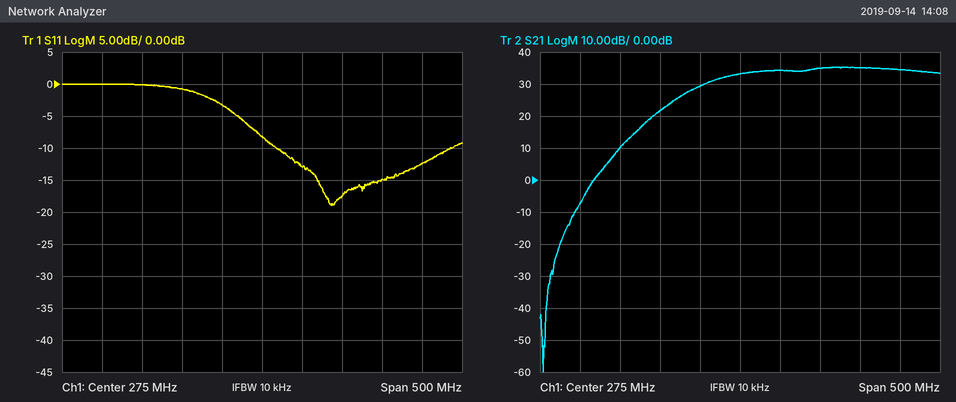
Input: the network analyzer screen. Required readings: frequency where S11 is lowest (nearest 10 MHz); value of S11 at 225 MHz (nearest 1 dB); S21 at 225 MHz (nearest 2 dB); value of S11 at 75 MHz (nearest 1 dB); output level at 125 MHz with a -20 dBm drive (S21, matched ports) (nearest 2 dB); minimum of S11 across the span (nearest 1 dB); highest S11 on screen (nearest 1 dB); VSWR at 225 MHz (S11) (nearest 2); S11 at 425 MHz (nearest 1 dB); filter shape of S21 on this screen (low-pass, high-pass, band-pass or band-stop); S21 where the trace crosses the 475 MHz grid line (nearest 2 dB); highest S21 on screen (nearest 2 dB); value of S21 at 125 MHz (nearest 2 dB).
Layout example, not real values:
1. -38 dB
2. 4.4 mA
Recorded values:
1. 360 MHz
2. -3 dB
3. 30 dB
4. 0 dB
5. -10 dBm
6. -19 dB
7. 0 dB
8. 6
9. -15 dB
10. high-pass
11. 34 dB
12. 36 dB
13. 10 dB
